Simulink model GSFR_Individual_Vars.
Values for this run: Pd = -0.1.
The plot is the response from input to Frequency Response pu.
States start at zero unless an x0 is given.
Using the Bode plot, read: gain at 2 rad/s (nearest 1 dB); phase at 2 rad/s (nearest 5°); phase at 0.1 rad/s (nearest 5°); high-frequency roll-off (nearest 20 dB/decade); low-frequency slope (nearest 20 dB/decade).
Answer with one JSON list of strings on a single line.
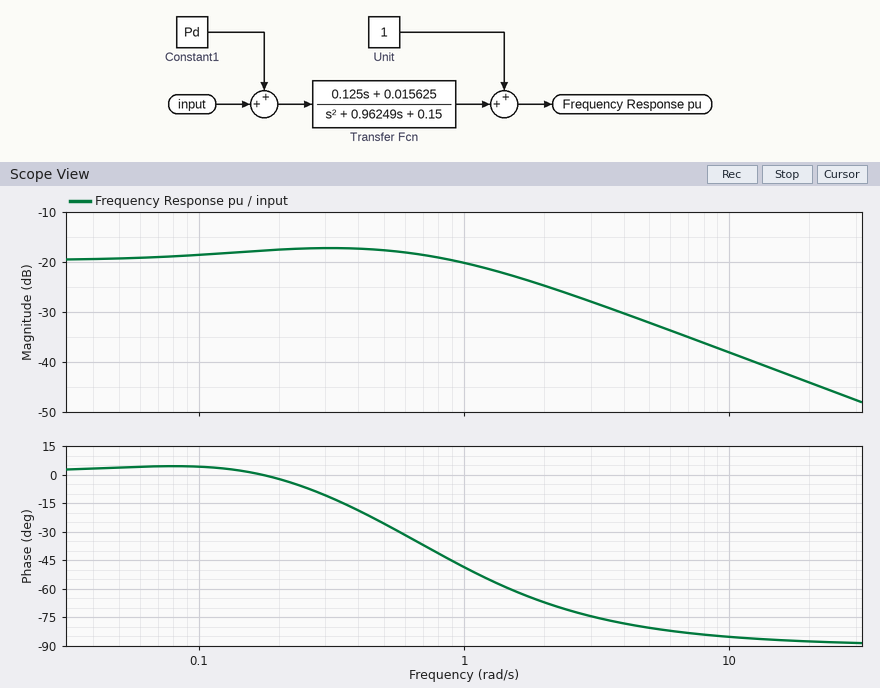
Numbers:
["-25 dB", "-65°", "5°", "-20 dB/decade", "0 dB/decade"]
